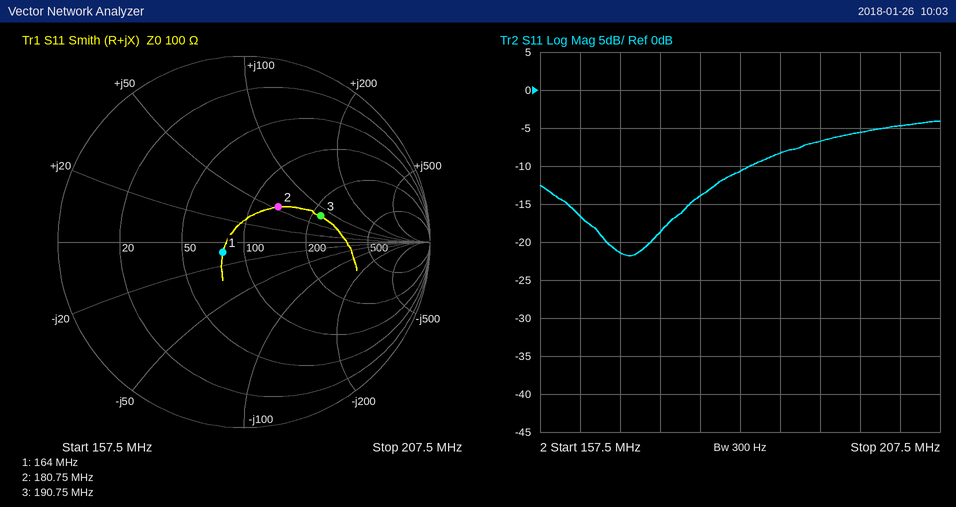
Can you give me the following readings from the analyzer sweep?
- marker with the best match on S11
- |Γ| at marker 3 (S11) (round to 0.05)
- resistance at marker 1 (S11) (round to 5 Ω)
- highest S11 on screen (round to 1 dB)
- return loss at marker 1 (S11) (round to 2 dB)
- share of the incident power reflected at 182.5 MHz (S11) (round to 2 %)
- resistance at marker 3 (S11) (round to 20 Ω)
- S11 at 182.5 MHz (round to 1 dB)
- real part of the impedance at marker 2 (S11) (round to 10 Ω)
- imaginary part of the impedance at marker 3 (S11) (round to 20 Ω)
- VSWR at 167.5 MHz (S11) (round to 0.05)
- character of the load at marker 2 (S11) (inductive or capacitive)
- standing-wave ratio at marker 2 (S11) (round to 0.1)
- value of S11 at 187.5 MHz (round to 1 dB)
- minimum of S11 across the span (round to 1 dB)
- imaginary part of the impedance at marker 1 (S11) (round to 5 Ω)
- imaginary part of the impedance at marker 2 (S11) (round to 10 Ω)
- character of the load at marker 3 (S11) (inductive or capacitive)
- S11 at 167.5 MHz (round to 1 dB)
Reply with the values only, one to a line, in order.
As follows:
marker 1
0.45
80 Ω
-4 dB
18 dB
8 %
220 Ω
-11 dB
130 Ω
+80 Ω
1.20
inductive
1.7
-8 dB
-22 dB
-10 Ω
+50 Ω
inductive
-21 dB
